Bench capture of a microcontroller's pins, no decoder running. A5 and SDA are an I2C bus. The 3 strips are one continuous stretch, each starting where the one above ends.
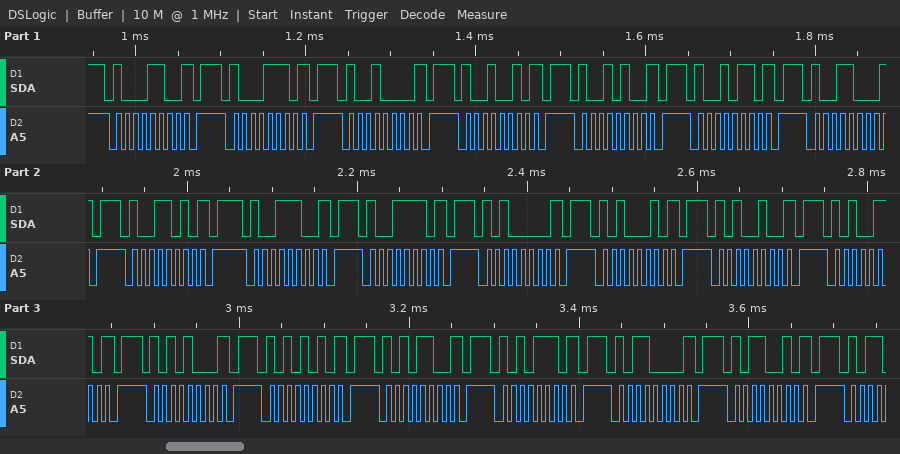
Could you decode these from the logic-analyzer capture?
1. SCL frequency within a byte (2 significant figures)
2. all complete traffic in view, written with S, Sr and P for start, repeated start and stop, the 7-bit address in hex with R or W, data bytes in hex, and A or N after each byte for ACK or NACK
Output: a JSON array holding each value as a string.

["100 kHz", "S 46W N P S 47W N P S 48W N P S 49W N P S 4AW N P S 4BW N P S 4CW N P S 4DW N P S 4EW N P S 4FW N P S 50W N P S 51W N P S 52W N P S 53W N P S 54W N P S 55W N P S 56W N P S 57W N P S 58W N P S 59W N P"]
